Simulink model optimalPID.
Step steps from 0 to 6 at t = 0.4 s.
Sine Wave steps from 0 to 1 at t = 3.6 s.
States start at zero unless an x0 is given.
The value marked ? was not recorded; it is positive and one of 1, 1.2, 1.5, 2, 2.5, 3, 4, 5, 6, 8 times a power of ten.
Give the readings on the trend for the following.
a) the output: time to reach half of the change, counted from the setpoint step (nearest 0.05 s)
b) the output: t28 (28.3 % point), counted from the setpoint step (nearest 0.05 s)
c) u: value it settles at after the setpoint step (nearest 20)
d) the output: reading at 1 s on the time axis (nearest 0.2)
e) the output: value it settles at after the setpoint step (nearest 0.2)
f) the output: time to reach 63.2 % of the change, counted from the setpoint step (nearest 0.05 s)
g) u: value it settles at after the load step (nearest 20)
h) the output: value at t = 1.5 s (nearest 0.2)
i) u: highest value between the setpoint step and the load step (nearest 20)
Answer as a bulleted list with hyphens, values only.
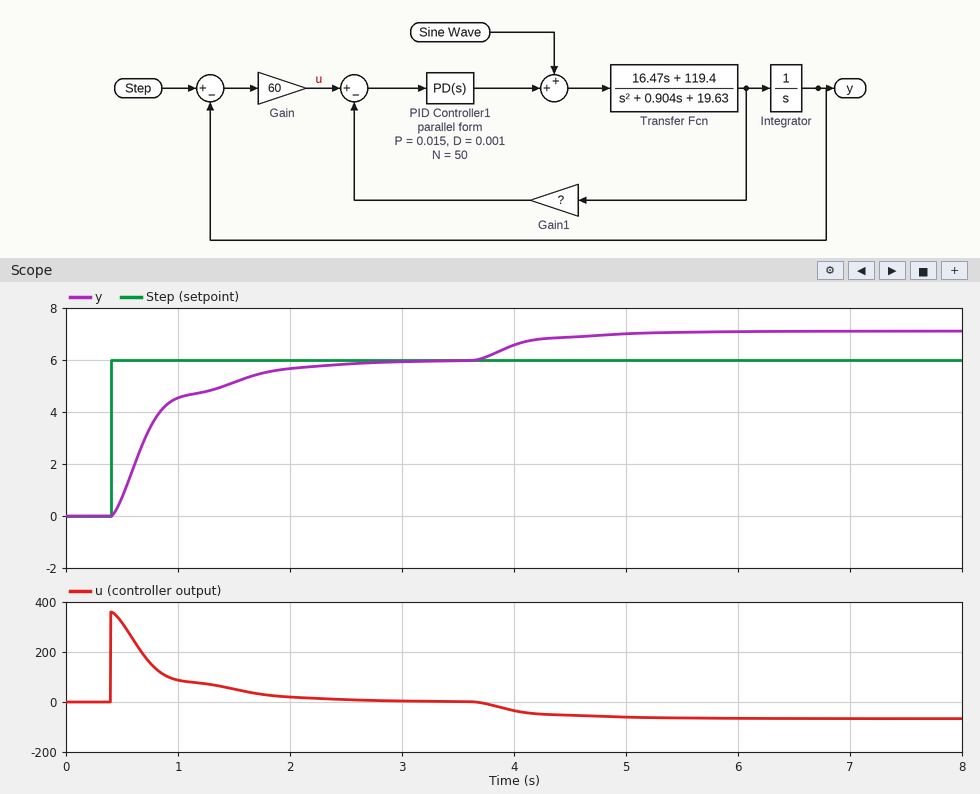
- 0.30 s
- 0.20 s
- 0
- 4.6
- 6.0
- 0.40 s
- -60
- 5.2
- 360
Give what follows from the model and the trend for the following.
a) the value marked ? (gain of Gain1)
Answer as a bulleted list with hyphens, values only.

- 20
